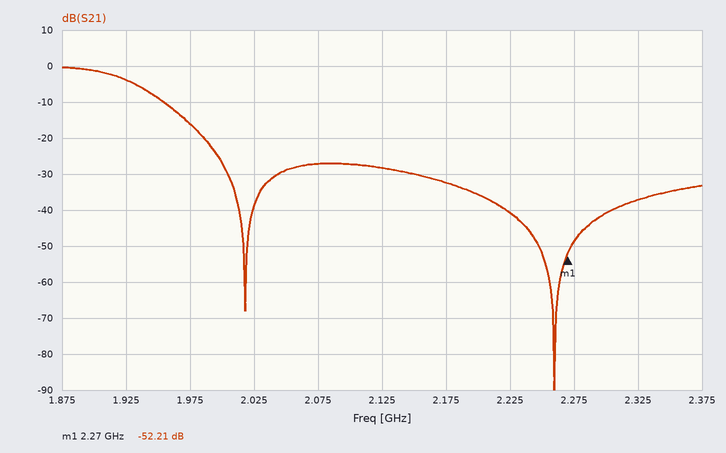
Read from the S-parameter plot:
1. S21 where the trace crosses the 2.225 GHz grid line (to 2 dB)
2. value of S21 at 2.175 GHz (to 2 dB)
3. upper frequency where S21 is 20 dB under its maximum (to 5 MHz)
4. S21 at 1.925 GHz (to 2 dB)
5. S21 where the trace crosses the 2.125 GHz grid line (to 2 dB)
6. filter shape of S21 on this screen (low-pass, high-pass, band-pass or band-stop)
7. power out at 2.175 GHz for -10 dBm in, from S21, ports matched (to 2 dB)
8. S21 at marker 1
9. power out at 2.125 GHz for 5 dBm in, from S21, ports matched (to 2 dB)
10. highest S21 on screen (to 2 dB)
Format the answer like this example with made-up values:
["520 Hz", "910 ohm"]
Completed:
["-40 dB", "-32 dB", "1.985 GHz", "-4 dB", "-28 dB", "low-pass", "-42 dBm", "-52.21 dB", "-24 dBm", "0 dB"]
